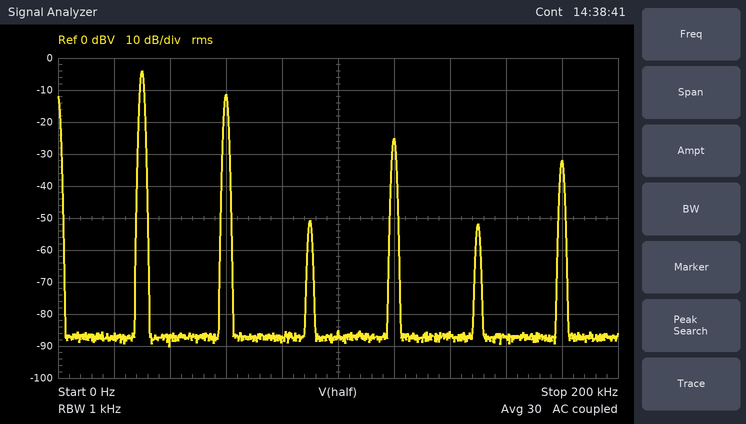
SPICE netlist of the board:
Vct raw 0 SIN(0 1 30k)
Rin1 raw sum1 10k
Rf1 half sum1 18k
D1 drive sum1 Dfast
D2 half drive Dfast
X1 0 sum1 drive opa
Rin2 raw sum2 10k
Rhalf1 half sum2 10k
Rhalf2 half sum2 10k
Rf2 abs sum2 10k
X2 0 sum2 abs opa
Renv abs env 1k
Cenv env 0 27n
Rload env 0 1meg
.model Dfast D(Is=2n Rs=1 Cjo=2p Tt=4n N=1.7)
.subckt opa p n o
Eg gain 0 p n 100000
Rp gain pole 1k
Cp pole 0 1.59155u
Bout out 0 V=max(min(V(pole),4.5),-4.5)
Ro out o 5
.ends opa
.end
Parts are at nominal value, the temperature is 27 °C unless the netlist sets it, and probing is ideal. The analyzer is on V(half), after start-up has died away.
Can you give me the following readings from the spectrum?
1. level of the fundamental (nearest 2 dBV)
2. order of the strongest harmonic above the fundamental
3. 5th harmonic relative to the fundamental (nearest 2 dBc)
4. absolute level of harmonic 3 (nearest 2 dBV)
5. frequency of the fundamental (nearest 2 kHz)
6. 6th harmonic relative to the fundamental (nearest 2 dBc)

-4 dBV
2
-48 dBc
-50 dBV
30 kHz
-28 dBc
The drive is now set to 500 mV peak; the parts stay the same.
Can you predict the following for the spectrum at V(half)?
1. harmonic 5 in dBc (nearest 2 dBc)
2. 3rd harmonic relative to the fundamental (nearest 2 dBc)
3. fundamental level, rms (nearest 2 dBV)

-42 dBc
-42 dBc
-10 dBV
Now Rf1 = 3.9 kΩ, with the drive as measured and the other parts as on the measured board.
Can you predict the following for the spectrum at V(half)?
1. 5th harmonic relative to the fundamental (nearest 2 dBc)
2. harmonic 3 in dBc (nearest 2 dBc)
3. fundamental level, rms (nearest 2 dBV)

-42 dBc
-42 dBc
-18 dBV
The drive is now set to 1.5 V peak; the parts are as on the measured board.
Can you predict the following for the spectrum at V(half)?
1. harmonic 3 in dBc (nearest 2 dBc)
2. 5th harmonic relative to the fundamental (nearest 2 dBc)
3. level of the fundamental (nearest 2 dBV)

-50 dBc
-50 dBc
0 dBV
